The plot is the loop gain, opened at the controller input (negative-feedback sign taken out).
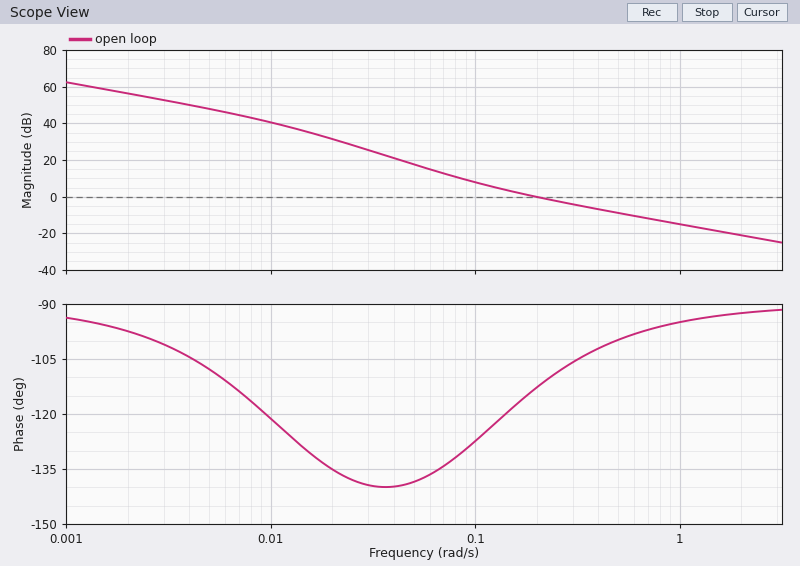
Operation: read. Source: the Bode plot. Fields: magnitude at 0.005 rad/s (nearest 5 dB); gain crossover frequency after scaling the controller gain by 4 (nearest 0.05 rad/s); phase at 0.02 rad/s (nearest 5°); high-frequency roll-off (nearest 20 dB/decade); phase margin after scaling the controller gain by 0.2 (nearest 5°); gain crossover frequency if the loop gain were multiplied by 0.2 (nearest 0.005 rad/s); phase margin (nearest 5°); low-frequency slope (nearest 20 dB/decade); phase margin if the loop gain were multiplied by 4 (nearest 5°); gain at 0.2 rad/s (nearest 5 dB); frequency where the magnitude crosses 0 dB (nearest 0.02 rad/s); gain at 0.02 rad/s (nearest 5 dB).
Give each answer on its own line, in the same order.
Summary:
50 dB
0.70 rad/s
-135°
-20 dB/decade
45°
0.065 rad/s
65°
-20 dB/decade
85°
0 dB
0.20 rad/s
30 dB
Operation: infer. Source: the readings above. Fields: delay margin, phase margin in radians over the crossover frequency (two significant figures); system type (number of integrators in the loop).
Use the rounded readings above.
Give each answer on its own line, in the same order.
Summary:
5.7 s
1
